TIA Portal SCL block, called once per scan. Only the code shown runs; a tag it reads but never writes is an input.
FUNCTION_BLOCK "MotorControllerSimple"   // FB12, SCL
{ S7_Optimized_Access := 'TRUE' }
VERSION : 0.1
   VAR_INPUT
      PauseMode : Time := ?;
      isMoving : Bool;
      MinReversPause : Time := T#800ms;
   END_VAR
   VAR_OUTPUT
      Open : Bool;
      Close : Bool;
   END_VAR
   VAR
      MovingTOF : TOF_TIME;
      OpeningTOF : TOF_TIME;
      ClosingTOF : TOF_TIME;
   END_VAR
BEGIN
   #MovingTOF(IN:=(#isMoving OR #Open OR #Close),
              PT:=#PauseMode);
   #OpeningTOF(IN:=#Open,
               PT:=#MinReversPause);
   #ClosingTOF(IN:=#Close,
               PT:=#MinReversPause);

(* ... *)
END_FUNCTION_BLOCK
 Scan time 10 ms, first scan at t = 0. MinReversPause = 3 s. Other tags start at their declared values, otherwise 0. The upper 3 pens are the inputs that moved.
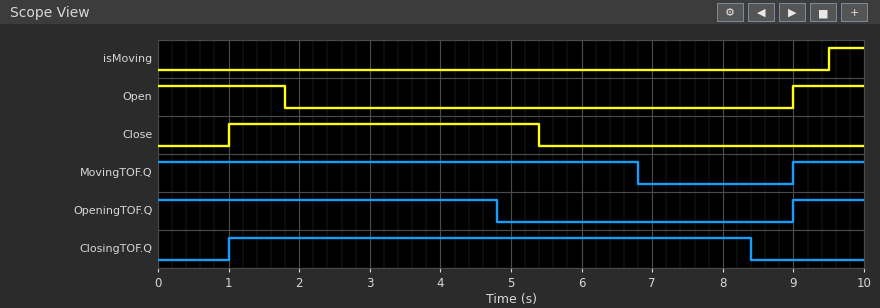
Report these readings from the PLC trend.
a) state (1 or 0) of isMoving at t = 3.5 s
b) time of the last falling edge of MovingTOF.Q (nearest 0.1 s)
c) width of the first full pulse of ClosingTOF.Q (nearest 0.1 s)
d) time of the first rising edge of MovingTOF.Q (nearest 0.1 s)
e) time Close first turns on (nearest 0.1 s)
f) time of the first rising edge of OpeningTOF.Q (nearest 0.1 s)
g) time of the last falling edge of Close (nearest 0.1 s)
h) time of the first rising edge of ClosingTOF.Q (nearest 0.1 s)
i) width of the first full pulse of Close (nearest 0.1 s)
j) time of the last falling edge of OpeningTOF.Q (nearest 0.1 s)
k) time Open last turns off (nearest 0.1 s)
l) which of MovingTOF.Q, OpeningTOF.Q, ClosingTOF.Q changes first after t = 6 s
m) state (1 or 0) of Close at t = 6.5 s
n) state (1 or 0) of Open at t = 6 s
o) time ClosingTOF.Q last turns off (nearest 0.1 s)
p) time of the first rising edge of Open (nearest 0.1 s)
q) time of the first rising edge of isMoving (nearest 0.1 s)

0
6.8 s
7.4 s
9.0 s
1.0 s
9.0 s
5.4 s
1.0 s
4.4 s
4.8 s
1.8 s
MovingTOF.Q
0
0
8.4 s
9.0 s
9.5 s
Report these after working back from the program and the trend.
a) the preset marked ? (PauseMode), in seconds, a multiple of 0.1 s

1.4 s
